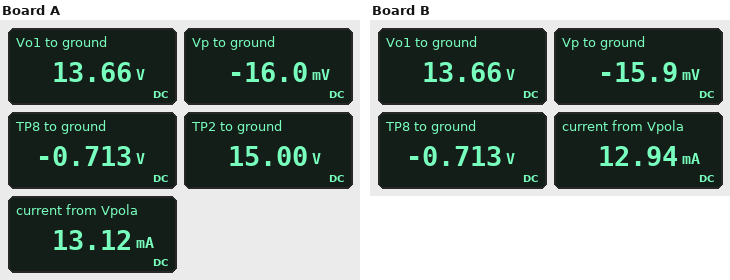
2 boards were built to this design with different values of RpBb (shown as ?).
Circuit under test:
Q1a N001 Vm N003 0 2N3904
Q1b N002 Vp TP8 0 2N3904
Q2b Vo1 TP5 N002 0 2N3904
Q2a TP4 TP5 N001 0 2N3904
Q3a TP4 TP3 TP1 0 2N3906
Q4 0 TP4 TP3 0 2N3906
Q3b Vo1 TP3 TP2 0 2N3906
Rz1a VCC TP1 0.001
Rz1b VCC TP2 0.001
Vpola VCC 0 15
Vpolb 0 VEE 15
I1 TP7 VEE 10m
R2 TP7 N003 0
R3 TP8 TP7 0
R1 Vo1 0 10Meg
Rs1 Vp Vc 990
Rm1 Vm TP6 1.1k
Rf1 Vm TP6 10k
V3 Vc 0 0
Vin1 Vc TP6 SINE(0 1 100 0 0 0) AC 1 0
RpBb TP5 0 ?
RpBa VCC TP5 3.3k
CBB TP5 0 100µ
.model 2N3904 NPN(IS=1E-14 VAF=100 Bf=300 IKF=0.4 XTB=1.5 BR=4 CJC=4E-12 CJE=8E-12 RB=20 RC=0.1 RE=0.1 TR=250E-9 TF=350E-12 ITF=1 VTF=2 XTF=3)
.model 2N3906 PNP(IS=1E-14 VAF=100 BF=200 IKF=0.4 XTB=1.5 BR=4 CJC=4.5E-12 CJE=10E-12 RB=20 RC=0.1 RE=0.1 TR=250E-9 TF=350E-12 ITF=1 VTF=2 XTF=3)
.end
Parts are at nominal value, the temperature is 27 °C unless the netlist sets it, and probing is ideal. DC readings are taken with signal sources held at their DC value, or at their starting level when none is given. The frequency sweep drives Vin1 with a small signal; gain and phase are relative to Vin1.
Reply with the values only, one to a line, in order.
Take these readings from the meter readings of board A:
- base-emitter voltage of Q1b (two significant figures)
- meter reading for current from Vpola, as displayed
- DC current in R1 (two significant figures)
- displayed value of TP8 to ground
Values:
700 mV
13.12 mA
1.4 µA
-0.713 V
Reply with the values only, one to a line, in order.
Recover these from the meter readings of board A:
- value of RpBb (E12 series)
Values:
1.5 kΩ
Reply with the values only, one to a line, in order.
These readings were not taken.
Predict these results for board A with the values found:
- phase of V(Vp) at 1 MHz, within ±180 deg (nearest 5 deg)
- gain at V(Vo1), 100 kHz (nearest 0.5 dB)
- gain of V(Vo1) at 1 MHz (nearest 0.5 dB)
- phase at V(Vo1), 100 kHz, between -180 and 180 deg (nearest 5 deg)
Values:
-160 deg
67.0 dB
58.5 dB
165 deg
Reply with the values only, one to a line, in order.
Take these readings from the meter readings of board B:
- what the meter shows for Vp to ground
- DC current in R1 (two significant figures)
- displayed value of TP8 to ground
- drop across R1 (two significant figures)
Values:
-15.9 mV
1.4 µA
-0.713 V
14 V
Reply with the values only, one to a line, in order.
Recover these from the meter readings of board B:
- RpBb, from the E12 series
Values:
1.8 kΩ
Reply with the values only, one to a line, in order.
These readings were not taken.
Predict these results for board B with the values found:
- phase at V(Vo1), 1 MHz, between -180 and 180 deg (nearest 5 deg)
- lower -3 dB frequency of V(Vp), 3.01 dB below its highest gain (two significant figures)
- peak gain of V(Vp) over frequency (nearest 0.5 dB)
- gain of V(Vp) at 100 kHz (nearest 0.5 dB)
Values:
95 deg
2.3 MHz
-6.5 dB
-14.5 dB
